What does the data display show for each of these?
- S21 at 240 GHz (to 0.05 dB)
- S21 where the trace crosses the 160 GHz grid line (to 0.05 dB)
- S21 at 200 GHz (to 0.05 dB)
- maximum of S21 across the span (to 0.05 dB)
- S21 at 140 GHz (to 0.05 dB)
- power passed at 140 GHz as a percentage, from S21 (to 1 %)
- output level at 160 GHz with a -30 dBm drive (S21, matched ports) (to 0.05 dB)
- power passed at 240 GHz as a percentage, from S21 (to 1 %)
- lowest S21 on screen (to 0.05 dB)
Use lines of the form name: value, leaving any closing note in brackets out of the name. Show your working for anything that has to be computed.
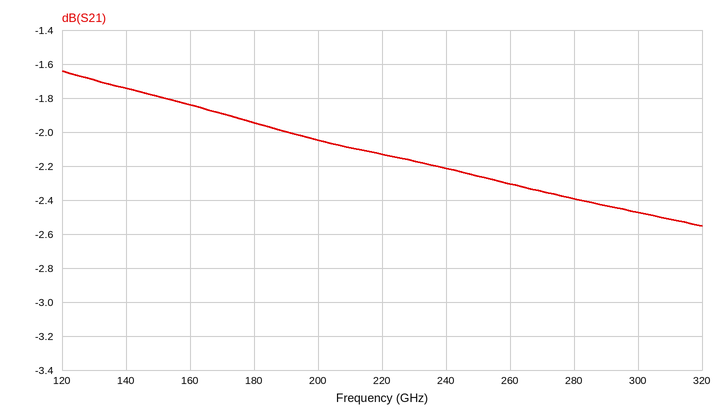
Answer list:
S21 at 240 GHz: -2.20 dB
S21 where the trace crosses the 160 GHz grid line: -1.85 dB
S21 at 200 GHz: -2.05 dB
maximum of S21 across the span: -1.65 dB
S21 at 140 GHz: -1.75 dB
power passed at 140 GHz as a percentage, from S21: 10^(-1.75/10) ≈ 67 %
output level at 160 GHz with a -30 dBm drive (S21, matched ports): -30 dBm + (-1.85 dB) = -31.85 dBm
power passed at 240 GHz as a percentage, from S21: 10^(-2.2/10) ≈ 60 %
lowest S21 on screen: -2.55 dB
